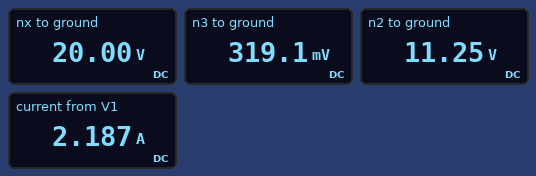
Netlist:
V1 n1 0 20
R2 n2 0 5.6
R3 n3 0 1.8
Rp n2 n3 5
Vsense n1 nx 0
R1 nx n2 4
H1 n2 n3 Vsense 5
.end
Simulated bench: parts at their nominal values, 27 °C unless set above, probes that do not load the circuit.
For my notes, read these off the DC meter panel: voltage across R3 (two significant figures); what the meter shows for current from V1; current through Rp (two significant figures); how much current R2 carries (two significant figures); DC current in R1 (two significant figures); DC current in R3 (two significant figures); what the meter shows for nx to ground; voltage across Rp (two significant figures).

320 mV
2.187 A
2.2 A
2.0 A
2.2 A
180 mA
20.00 V
11 V
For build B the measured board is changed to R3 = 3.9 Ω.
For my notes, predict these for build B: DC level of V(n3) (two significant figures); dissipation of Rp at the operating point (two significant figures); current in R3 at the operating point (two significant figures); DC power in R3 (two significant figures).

530 mV
23 W
140 mA
73 mW
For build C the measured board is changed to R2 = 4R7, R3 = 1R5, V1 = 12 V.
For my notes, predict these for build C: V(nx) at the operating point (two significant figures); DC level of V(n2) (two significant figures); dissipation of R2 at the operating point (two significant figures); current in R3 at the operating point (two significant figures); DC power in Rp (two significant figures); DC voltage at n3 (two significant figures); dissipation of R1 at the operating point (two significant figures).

12 V
6.6 V
9.3 W
65 mA
9.0 W
-98 mV
7.2 W
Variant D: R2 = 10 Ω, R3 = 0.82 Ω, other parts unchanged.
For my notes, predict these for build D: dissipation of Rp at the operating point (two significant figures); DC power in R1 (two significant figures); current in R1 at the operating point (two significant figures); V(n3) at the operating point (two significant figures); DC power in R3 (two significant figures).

23 W
18 W
2.1 A
810 mV
800 mW
